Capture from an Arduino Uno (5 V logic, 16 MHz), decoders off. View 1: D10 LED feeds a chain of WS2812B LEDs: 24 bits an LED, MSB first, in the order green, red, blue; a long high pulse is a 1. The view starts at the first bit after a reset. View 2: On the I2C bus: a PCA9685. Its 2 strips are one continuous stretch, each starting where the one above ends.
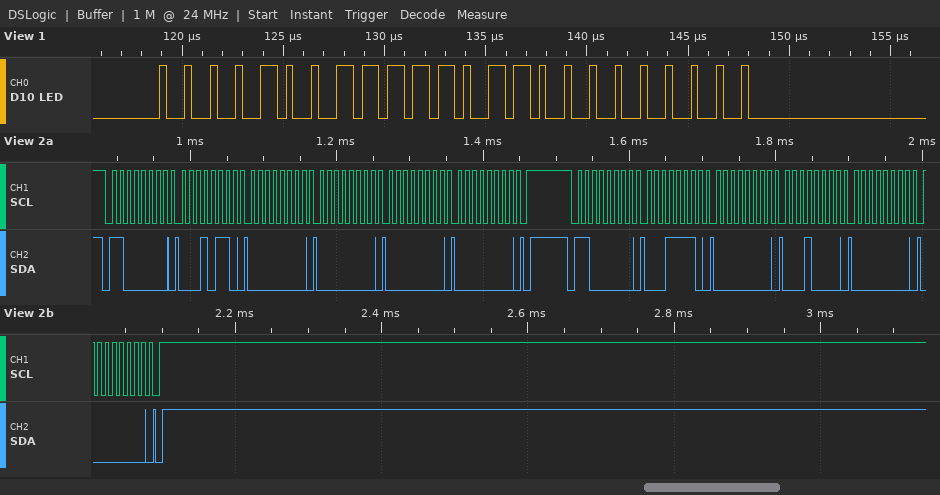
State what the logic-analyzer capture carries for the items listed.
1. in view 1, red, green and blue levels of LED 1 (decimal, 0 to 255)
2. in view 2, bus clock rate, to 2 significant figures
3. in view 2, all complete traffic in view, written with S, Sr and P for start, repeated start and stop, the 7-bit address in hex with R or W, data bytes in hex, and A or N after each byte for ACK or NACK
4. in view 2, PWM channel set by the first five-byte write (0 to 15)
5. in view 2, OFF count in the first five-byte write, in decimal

246, 9, 0
100 kHz
S 60W A 16 A 00 A 00 A 00 A 00 A P S 60W A 1E A 00 A 10 A 00 A 00 A P
4
0
